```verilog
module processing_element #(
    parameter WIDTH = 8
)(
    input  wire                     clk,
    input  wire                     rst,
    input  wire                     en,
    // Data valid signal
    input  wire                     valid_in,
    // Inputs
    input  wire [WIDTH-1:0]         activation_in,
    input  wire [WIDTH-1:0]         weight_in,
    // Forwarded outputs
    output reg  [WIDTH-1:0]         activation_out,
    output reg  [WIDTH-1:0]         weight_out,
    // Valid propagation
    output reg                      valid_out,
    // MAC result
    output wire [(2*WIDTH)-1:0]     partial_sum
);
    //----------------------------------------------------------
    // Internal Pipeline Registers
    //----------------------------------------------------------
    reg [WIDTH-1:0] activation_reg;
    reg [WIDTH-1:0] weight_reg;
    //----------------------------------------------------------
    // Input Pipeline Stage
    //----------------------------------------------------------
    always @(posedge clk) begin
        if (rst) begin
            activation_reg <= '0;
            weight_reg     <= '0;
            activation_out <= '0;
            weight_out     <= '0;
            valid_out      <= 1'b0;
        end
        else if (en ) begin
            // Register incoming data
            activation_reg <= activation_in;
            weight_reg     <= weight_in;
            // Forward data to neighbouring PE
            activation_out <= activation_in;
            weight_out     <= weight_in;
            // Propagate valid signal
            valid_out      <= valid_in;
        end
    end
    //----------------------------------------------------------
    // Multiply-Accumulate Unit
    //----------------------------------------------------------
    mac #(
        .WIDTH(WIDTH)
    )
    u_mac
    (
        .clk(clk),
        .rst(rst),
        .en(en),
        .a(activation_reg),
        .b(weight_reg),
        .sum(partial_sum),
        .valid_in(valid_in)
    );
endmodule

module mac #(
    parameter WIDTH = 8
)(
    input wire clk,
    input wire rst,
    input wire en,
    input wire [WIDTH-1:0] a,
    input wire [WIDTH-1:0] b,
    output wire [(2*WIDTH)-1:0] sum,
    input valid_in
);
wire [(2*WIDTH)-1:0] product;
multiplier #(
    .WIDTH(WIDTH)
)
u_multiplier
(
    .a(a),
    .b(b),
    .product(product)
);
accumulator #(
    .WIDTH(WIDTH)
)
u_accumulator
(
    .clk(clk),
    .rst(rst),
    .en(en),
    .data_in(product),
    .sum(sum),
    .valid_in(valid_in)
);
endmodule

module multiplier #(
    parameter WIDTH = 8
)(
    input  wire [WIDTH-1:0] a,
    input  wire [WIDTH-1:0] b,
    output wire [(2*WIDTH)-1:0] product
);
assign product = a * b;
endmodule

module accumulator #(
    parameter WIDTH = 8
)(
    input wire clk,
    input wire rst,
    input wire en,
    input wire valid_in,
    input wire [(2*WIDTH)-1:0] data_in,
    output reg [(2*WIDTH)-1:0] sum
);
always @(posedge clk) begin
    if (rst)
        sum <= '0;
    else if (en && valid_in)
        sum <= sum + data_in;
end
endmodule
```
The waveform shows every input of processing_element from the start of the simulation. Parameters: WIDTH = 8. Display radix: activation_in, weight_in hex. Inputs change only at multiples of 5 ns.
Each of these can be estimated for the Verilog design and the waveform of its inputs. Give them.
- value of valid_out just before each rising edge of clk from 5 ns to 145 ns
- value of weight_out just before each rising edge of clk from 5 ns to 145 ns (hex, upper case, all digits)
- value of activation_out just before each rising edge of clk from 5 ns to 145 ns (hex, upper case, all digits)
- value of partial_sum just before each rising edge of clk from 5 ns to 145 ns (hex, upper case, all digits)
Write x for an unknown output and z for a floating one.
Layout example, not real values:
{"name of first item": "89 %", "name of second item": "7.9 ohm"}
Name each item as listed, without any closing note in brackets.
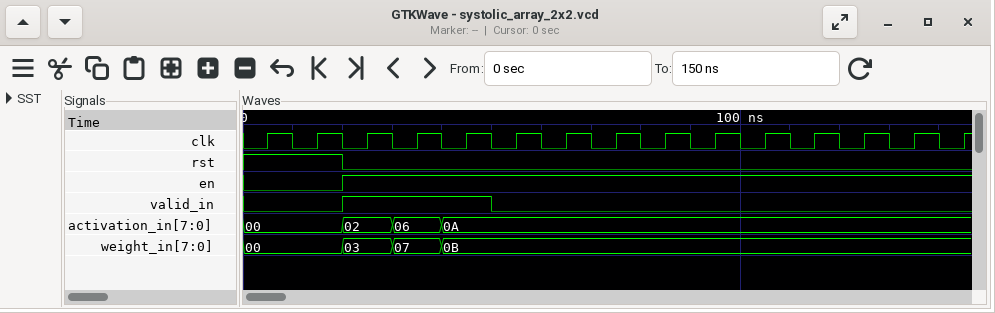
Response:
{"value of valid_out just before each rising edge of clk from 5 ns to 145 ns": "x 0 0 1 1 1 0 0 0 0 0 0 0 0 0", "value of weight_out just before each rising edge of clk from 5 ns to 145 ns": "x, 00, 00, 03, 07, 0B, 0B, 0B, 0B, 0B, 0B, 0B, 0B, 0B, 0B", "value of activation_out just before each rising edge of clk from 5 ns to 145 ns": "x, 00, 00, 02, 06, 0A, 0A, 0A, 0A, 0A, 0A, 0A, 0A, 0A, 0A", "value of partial_sum just before each rising edge of clk from 5 ns to 145 ns": "x, 0000, 0000, 0000, 0006, 0030, 0030, 0030, 0030, 0030, 0030, 0030, 0030, 0030, 0030"}
